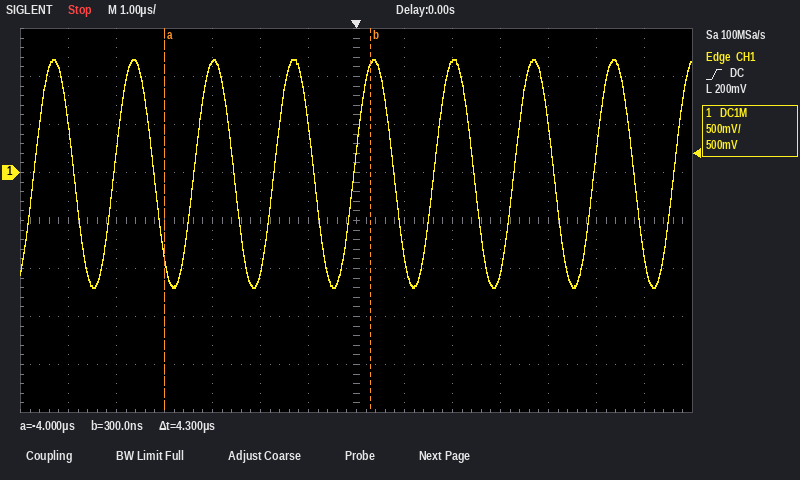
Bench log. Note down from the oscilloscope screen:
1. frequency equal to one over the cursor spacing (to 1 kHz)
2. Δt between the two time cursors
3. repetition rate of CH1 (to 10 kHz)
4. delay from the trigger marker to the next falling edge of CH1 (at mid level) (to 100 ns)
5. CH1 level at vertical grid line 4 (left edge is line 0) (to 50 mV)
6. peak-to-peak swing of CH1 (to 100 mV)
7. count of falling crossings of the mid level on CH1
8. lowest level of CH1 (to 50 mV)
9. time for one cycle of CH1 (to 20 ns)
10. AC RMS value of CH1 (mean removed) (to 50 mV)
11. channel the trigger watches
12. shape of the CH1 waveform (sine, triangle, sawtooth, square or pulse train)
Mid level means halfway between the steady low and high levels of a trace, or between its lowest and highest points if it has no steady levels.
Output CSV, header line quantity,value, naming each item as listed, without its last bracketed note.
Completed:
quantity,value
frequency equal to one over the cursor spacing,233 kHz
Δt between the two time cursors,4.3 µs
repetition rate of CH1,600 kHz
delay from the trigger marker to the next falling edge of CH1 (at mid level),800 ns
CH1 level at vertical grid line 4 (left edge is line 0),1.15 V
peak-to-peak swing of CH1,2.40 V
count of falling crossings of the mid level on CH1,8
lowest level of CH1,-1.20 V
time for one cycle of CH1,1.66 µs
AC RMS value of CH1 (mean removed),850 mV
channel the trigger watches,CH1
shape of the CH1 waveform,sine
